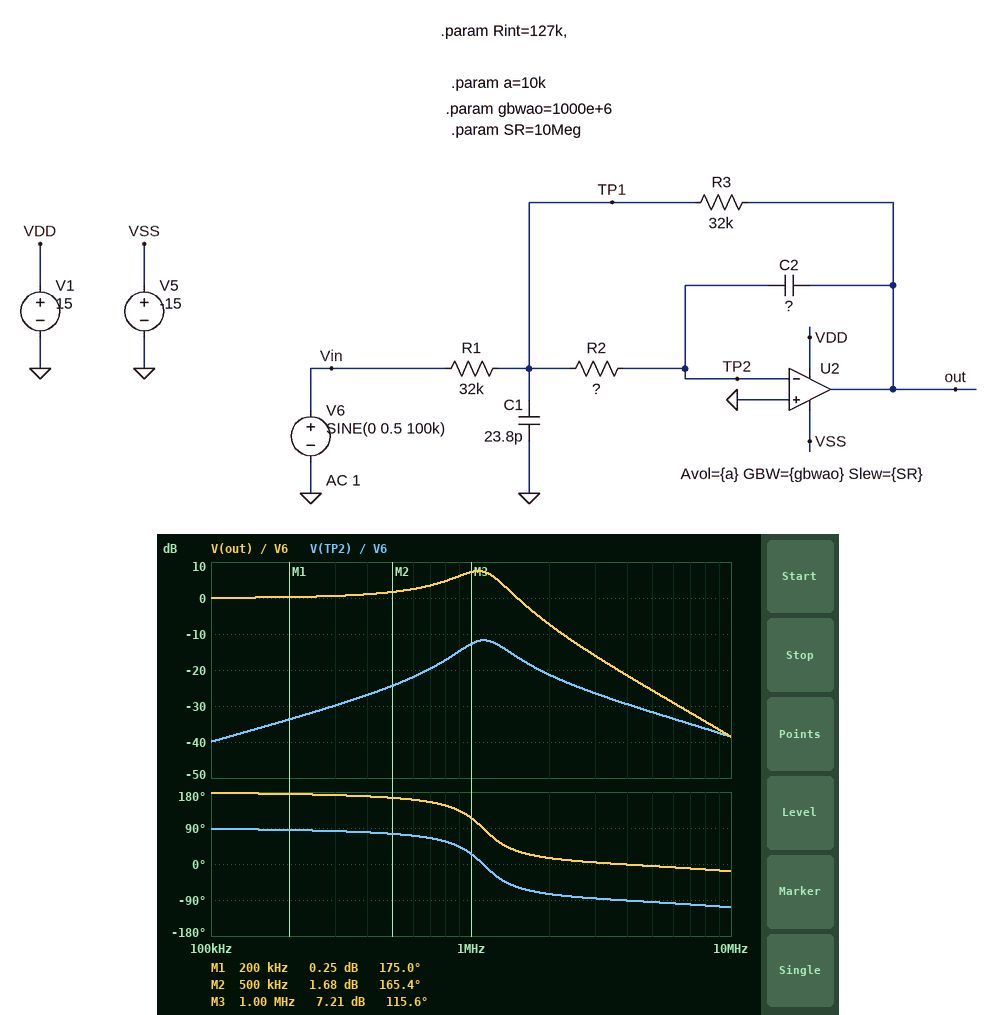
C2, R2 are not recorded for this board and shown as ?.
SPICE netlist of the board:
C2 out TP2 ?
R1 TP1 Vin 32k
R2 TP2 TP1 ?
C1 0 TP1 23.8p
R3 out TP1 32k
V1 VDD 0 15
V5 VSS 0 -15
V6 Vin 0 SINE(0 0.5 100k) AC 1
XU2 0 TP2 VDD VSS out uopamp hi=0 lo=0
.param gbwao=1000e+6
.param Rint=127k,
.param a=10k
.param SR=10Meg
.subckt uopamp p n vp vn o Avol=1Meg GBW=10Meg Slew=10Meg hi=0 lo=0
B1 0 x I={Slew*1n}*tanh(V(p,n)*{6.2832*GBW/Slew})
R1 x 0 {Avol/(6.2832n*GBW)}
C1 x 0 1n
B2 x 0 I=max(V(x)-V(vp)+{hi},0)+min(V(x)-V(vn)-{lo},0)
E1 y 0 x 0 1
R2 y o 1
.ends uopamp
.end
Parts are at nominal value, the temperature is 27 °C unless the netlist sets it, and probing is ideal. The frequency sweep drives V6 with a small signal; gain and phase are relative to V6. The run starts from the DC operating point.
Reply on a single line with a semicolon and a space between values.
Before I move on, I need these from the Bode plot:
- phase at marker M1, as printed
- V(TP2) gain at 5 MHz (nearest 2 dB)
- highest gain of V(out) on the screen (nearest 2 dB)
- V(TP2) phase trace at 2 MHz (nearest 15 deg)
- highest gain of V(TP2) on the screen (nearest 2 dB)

175.0 deg; -32 dB; 8 dB; -75 deg; -12 dB
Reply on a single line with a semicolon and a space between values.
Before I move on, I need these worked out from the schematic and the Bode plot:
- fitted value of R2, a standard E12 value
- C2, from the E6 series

22 kΩ; 470 fF
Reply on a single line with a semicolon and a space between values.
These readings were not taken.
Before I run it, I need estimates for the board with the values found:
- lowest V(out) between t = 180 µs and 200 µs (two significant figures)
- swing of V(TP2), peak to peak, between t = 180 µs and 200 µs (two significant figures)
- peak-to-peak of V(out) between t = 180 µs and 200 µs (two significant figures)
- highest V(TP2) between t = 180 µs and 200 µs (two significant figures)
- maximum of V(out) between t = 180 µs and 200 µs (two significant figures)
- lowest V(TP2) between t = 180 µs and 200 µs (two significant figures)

-500 mV; 10 mV; 1.0 V; 5.0 mV; 500 mV; -5.0 mV
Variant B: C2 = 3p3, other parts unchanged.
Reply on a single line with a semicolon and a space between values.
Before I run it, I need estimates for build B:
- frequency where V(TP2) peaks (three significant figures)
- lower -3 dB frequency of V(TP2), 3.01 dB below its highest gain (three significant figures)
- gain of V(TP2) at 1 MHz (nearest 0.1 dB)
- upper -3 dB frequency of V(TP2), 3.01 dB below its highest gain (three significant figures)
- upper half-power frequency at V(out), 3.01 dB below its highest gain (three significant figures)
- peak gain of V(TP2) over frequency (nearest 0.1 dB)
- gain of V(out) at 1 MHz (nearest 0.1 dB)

610 kHz; 371 kHz; -27.6 dB; 1.00 MHz; 709 kHz; -24.6 dB; -7.6 dB
